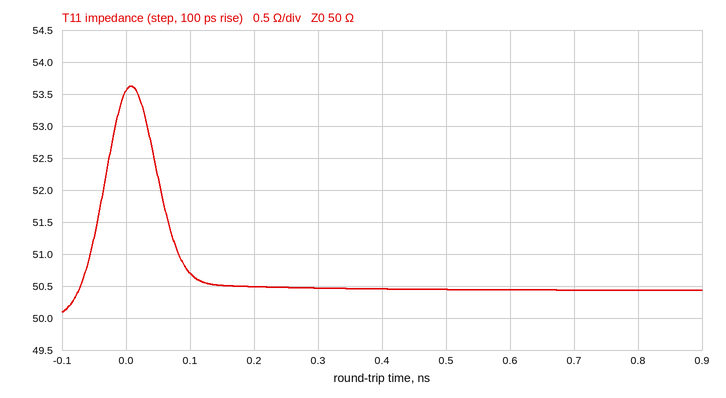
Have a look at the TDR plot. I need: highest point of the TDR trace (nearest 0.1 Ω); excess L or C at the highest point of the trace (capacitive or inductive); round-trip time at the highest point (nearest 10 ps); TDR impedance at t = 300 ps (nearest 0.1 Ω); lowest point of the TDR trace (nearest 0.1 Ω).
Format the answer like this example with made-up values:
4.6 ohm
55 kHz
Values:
53.6 Ω
inductive
10 ps
50.5 Ω
50.1 Ω
